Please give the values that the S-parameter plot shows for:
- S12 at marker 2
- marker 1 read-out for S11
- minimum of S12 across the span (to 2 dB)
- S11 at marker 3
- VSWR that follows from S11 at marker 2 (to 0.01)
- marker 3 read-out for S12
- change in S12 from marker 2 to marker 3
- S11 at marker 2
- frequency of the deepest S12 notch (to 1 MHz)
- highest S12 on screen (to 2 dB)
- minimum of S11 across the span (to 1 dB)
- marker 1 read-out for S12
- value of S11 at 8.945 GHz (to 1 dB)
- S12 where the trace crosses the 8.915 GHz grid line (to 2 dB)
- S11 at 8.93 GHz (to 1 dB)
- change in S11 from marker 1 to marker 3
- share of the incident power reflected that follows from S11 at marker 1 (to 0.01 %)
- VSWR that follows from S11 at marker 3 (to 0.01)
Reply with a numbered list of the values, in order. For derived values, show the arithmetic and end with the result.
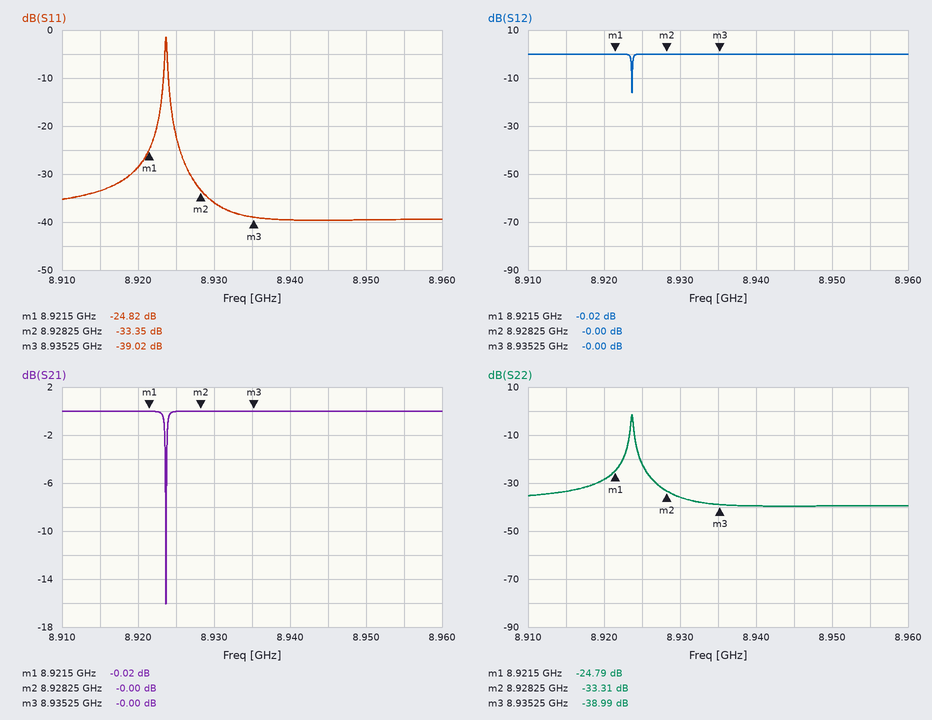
1. -0.00 dB
2. -24.82 dB
3. -16 dB
4. -39.02 dB
5. (1 + 0.0215)/(1 − 0.0215) ≈ 1.04
6. -0.00 dB
7. -0 − (-0) = 0.00 dB
8. -33.35 dB
9. 8.924 GHz
10. 0 dB
11. -40 dB
12. -0.02 dB
13. -40 dB
14. 0 dB
15. -36 dB
16. -39.02 − (-24.82) = -14.20 dB
17. 10^(-24.82/10) ≈ 0.33 %
18. (1 + 0.0112)/(1 − 0.0112) ≈ 1.02
